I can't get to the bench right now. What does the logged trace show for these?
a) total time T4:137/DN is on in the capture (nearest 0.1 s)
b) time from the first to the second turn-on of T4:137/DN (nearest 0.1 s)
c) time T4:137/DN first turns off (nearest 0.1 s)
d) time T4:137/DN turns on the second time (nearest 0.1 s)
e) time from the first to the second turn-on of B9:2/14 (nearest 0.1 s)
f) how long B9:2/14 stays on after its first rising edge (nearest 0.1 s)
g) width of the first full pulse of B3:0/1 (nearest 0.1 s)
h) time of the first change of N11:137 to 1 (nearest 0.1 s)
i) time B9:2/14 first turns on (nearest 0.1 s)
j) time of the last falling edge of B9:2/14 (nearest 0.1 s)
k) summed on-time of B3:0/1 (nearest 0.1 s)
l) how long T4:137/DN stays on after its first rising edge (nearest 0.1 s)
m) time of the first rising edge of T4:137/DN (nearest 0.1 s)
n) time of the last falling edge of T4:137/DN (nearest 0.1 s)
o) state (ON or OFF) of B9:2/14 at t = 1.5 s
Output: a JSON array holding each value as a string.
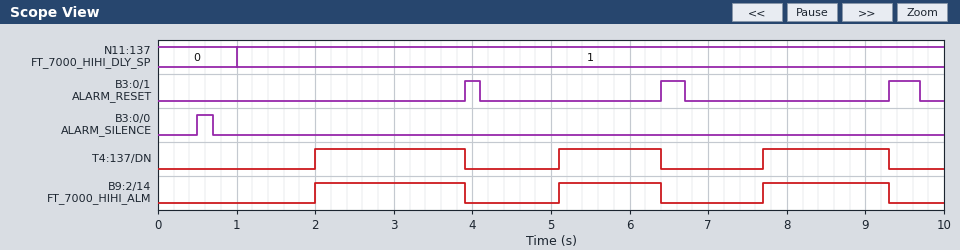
["4.8 s", "3.1 s", "3.9 s", "5.1 s", "3.1 s", "1.9 s", "0.2 s", "1.0 s", "2.0 s", "9.3 s", "0.9 s", "1.9 s", "2.0 s", "9.3 s", "OFF"]
